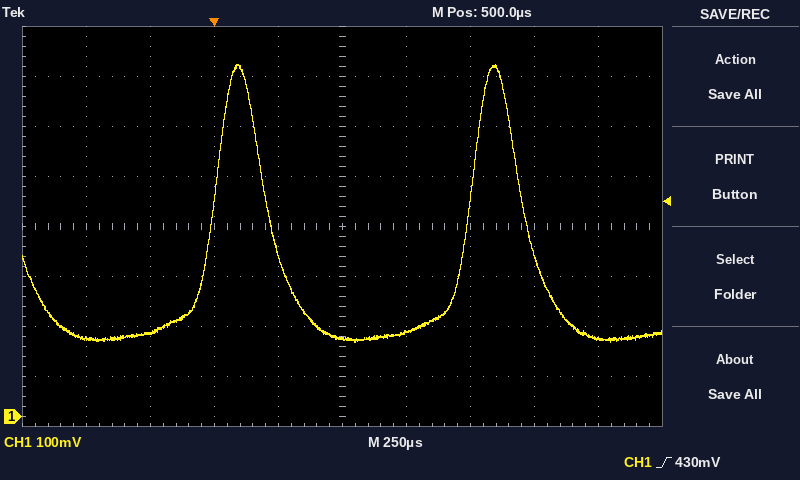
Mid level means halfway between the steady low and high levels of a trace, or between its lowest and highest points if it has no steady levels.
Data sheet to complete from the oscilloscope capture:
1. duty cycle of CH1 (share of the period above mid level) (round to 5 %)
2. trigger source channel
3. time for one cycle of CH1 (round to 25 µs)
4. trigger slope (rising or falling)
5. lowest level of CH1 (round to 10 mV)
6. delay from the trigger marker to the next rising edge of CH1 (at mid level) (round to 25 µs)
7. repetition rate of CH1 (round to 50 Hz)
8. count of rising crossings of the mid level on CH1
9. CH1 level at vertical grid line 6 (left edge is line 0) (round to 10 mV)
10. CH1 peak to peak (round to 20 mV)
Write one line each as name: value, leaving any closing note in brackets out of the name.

duty cycle of CH1 (share of the period above mid level): 20 %
trigger source channel: CH1
time for one cycle of CH1: 1.000 ms
trigger slope: rising
lowest level of CH1: 150 mV
delay from the trigger marker to the next rising edge of CH1 (at mid level): 1.000 ms
repetition rate of CH1: 1.00 kHz
count of rising crossings of the mid level on CH1: 2
CH1 level at vertical grid line 6 (left edge is line 0): 170 mV
CH1 peak to peak: 560 mV
